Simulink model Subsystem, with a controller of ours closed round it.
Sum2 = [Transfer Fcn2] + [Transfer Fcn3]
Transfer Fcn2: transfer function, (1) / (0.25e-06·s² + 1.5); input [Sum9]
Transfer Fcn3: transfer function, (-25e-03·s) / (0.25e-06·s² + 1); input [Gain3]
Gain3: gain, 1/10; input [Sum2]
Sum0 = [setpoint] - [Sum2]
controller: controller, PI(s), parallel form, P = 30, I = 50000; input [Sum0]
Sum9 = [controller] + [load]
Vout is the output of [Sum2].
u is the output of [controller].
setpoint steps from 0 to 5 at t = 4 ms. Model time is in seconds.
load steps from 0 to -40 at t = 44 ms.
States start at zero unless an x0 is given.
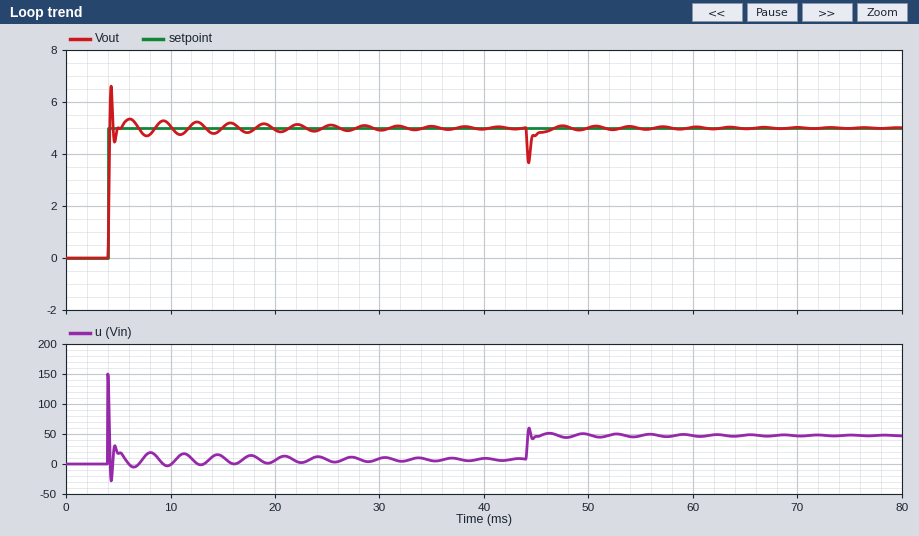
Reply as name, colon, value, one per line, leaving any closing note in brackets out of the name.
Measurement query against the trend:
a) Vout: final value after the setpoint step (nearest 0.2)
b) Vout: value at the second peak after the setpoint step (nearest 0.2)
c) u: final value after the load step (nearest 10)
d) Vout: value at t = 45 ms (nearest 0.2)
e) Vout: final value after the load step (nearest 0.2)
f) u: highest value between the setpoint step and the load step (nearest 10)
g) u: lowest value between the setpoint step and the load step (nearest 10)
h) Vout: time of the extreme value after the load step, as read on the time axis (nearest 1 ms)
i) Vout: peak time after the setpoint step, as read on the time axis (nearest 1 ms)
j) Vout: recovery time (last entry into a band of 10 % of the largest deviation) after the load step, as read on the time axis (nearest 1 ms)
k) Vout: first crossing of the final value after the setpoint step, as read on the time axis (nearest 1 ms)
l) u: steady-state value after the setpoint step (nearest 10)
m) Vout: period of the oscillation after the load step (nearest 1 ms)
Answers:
Vout: final value after the setpoint step: 5.0
Vout: value at the second peak after the setpoint step: 5.4
u: final value after the load step: 50
Vout: value at t = 45 ms: 4.8
Vout: final value after the load step: 5.0
u: highest value between the setpoint step and the load step: 150
u: lowest value between the setpoint step and the load step: -30
Vout: time of the extreme value after the load step, as read on the time axis: 44 ms
Vout: peak time after the setpoint step, as read on the time axis: 4 ms
Vout: recovery time (last entry into a band of 10 % of the largest deviation) after the load step, as read on the time axis: 46 ms
Vout: first crossing of the final value after the setpoint step, as read on the time axis: 4 ms
u: steady-state value after the setpoint step: 10
Vout: period of the oscillation after the load step: 5 ms
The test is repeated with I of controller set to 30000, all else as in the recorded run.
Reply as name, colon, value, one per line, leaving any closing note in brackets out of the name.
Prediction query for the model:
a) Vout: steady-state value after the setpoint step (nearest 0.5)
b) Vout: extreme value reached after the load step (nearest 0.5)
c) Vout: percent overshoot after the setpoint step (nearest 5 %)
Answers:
Vout: steady-state value after the setpoint step: 5.0
Vout: extreme value reached after the load step: 3.5
Vout: percent overshoot after the setpoint step: 25 %
